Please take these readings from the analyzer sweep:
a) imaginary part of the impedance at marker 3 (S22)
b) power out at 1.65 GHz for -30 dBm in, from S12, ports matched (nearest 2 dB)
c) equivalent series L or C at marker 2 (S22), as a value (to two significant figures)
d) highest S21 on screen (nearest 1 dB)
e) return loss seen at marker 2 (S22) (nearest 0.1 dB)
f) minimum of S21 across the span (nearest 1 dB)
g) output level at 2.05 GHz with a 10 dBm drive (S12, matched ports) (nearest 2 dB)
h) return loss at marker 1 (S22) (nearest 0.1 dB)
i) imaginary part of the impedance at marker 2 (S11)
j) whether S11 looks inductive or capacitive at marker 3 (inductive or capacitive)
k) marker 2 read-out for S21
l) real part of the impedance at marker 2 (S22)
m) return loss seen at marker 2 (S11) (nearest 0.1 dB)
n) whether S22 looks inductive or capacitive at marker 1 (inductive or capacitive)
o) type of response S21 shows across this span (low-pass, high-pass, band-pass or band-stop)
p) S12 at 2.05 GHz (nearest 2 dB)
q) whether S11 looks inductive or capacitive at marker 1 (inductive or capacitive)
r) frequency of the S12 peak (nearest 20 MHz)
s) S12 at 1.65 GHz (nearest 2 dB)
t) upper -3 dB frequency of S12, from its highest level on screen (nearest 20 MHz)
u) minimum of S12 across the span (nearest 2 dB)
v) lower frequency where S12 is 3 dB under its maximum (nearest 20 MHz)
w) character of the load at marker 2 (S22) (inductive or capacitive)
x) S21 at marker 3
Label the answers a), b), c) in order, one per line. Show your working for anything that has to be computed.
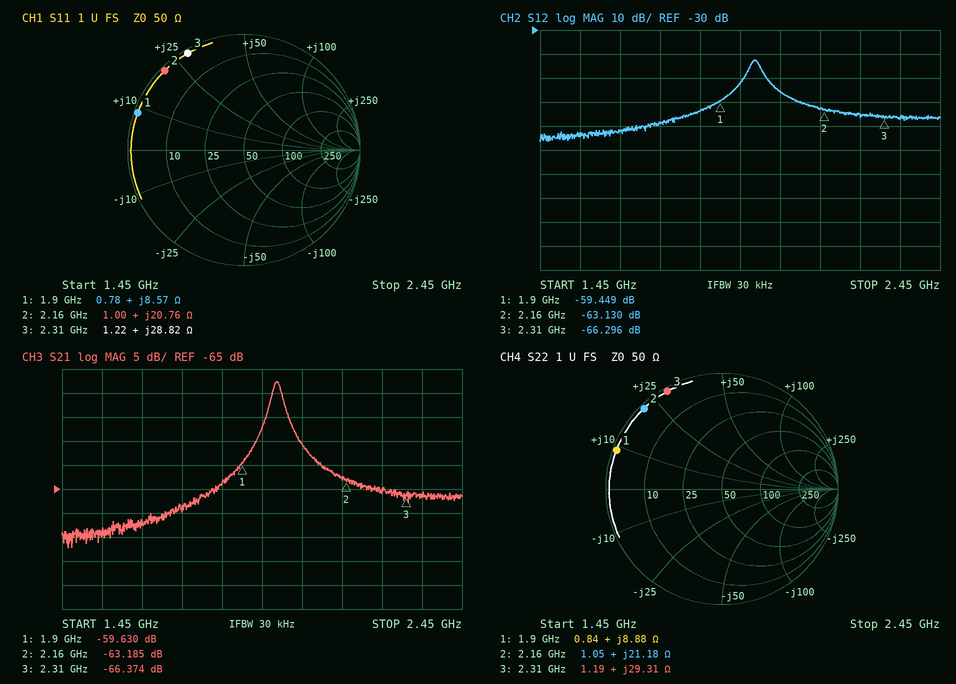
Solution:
a) +29.31 Ω
b) -30 dBm + (-72 dB) = -102 dBm
c) L = 21.18 Ω/(2π × 2.16 GHz) ≈ 1.6 nH
d) -43 dB
e) 0.3 dB
f) -77 dB
g) 10 dBm + (-56 dB) = -46 dBm
h) 0.3 dB
i) +20.76 Ω
j) inductive
k) -63.185 dB
l) 1.05 Ω
m) 0.3 dB
n) inductive
o) band-pass
p) -56 dB
q) inductive
r) 1.98 GHz
s) -72 dB
t) 2.00 GHz
u) -76 dB
v) 1.98 GHz
w) inductive
x) -66.374 dB
